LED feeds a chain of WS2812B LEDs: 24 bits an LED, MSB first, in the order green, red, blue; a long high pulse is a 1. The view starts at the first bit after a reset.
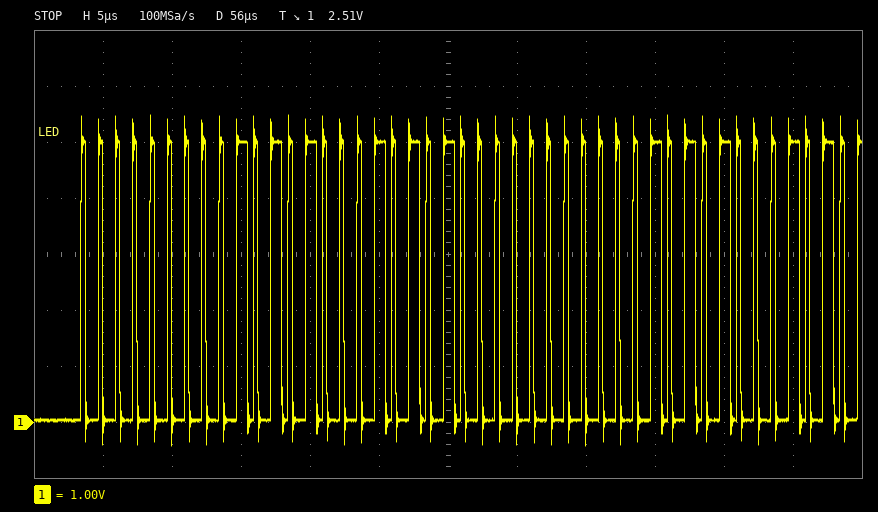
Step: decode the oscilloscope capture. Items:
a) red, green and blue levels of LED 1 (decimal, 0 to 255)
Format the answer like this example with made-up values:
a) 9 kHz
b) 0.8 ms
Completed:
a) 84, 0, 84
